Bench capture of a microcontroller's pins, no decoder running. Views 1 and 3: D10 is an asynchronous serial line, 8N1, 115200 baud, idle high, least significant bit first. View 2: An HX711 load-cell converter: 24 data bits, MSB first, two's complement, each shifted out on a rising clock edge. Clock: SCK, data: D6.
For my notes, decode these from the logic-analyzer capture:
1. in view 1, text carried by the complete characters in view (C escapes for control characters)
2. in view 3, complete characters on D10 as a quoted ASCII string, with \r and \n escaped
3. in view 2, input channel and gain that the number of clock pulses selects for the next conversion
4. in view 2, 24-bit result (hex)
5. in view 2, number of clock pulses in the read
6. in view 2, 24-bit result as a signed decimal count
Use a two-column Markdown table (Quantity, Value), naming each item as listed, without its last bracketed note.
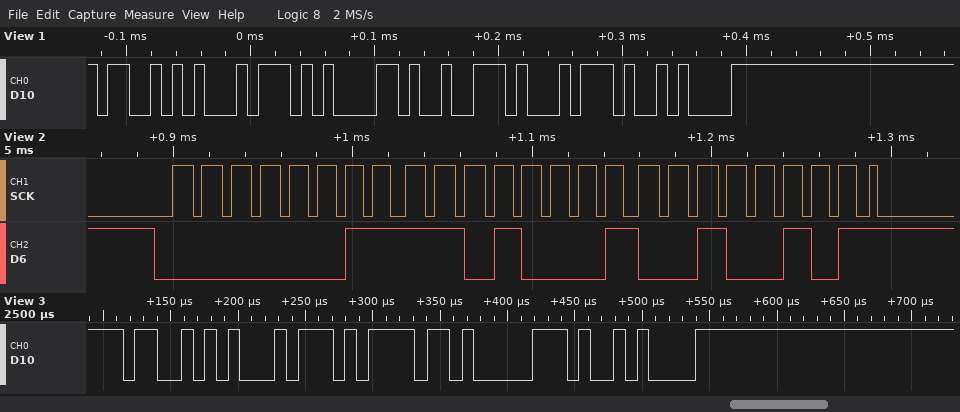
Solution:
| Quantity | Value |
|---|---|
| in view 1, text carried by the complete characters in view | "Start\n" |
| in view 3, complete characters on D10 as a quoted ASCII string, with \r and \n escaped | "Stop\n" |
| in view 2, input channel and gain that the number of clock pulses selects for the next conversion | channel A, gain 128 |
| in view 2, 24-bit result | 0x03D125 |
| in view 2, number of clock pulses in the read | 25 |
| in view 2, 24-bit result as a signed decimal count | 250149 |
